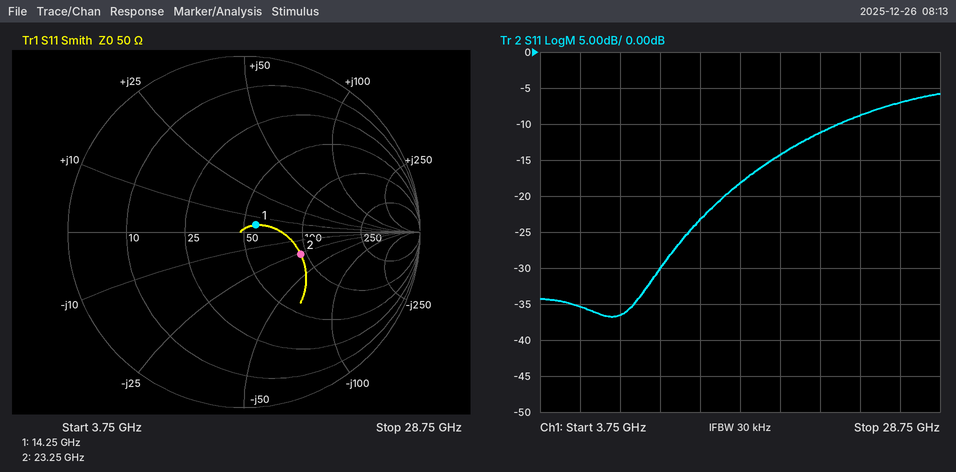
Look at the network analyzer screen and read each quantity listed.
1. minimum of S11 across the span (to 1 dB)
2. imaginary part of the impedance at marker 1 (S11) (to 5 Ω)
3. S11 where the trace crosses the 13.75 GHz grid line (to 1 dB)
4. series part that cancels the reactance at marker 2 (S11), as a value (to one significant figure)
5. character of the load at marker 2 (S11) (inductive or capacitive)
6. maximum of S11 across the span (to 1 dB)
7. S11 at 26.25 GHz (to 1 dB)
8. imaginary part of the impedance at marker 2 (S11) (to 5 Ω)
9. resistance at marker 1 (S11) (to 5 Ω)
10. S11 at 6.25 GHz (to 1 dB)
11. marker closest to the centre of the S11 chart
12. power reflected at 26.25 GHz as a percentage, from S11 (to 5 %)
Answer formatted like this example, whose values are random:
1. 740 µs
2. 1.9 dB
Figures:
1. -37 dB
2. +5 Ω
3. -23 dB
4. 200 pH
5. capacitive
6. -6 dB
7. -7 dB
8. -25 Ω
9. 55 Ω
10. -35 dB
11. marker 1
12. 20 %
